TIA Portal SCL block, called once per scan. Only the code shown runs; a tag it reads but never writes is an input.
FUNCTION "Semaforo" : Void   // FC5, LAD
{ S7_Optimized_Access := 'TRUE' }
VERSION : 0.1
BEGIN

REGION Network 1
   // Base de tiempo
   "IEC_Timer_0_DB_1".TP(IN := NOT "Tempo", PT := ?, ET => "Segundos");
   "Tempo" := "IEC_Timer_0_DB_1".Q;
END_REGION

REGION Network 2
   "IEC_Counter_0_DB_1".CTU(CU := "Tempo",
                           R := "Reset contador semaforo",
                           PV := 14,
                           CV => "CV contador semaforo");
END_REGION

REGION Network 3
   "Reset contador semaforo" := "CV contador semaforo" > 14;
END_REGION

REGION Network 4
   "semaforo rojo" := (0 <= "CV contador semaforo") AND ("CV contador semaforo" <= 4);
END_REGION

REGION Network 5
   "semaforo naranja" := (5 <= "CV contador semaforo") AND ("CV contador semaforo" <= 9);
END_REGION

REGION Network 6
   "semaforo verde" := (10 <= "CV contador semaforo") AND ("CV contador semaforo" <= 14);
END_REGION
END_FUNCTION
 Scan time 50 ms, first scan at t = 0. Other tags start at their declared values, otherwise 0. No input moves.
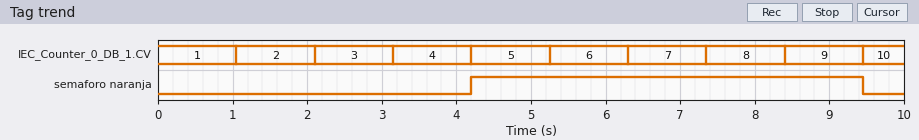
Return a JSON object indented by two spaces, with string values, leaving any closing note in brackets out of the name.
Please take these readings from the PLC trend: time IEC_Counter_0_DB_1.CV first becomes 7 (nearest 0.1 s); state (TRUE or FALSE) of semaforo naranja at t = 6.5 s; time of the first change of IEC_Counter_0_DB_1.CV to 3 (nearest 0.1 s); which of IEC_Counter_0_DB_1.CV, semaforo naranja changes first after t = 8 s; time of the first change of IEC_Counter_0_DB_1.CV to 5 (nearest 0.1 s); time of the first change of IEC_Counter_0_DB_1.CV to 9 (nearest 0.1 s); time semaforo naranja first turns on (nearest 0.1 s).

{
  "time IEC_Counter_0_DB_1.CV first becomes 7": "6.3 s",
  "state (TRUE or FALSE) of semaforo naranja at t = 6.5 s": "TRUE",
  "time of the first change of IEC_Counter_0_DB_1.CV to 3": "2.1 s",
  "which of IEC_Counter_0_DB_1.CV, semaforo naranja changes first after t = 8 s": "IEC_Counter_0_DB_1.CV",
  "time of the first change of IEC_Counter_0_DB_1.CV to 5": "4.2 s",
  "time of the first change of IEC_Counter_0_DB_1.CV to 9": "8.4 s",
  "time semaforo naranja first turns on": "4.2 s"
}
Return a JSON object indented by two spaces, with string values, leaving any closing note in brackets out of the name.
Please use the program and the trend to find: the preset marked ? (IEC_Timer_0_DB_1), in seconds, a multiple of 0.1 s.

{
  "the preset marked ? (IEC_Timer_0_DB_1), in seconds, a multiple of 0.1 s": "1.0 s"
}
